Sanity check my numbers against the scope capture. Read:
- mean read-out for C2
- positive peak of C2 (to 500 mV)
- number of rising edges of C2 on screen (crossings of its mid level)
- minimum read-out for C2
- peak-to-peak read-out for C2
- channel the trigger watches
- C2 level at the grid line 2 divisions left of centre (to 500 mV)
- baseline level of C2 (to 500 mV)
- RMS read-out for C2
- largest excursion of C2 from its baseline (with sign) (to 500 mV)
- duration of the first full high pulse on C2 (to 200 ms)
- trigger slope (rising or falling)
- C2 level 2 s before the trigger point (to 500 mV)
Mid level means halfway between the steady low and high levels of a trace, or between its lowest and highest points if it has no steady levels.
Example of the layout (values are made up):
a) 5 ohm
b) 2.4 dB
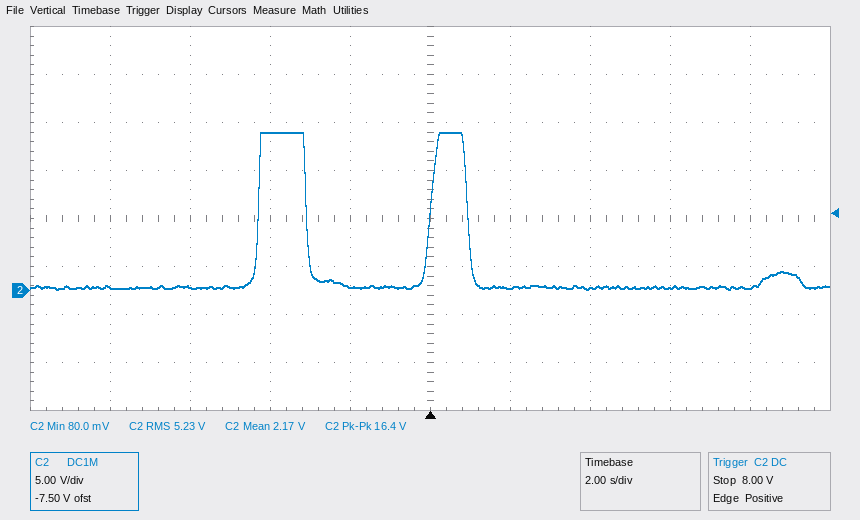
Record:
a) 2.17 V
b) 16.5 V
c) 2
d) 80.0 mV
e) 16.4 V
f) C2
g) 16.5 V
h) 500 mV
i) 5.23 V
j) +16.0 V
k) 1.2 s
l) rising
m) 500 mV
